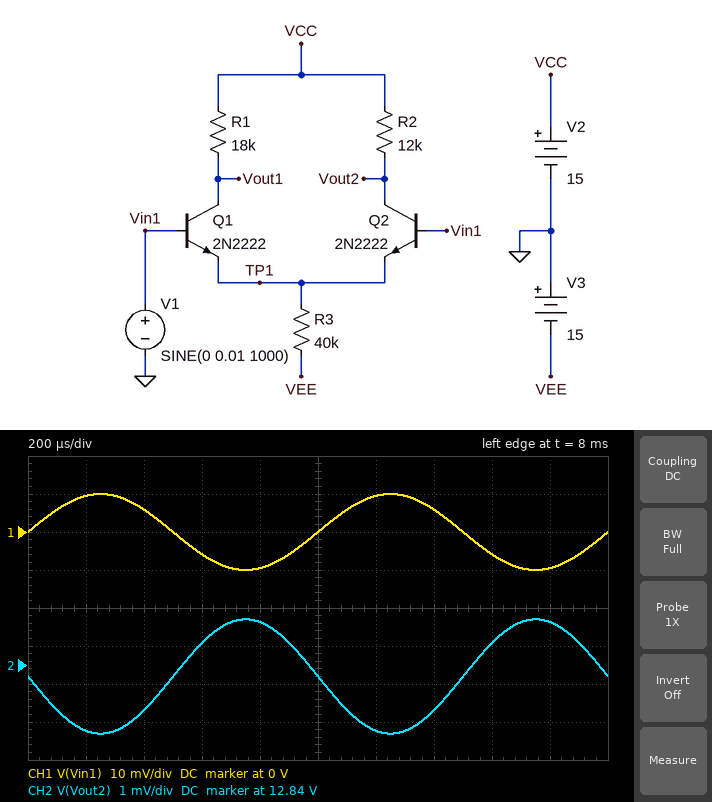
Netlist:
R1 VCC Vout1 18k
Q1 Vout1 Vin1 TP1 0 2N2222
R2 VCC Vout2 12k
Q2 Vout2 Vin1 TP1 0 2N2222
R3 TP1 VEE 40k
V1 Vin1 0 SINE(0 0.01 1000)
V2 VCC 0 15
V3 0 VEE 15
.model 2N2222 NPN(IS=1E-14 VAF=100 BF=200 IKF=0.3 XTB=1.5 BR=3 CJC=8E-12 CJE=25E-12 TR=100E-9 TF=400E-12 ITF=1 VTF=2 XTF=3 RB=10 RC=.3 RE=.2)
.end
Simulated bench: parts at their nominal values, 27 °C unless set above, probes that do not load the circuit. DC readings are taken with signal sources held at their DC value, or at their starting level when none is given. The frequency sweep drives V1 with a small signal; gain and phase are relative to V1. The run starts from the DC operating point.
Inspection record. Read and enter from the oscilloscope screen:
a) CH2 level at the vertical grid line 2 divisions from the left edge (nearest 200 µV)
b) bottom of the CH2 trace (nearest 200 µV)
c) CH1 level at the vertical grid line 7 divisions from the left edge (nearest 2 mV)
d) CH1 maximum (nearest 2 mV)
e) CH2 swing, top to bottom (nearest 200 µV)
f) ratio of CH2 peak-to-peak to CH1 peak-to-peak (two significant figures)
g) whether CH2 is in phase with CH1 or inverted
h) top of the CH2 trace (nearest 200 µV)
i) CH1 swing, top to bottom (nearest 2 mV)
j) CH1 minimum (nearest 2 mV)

12.8398 V
12.8392 V
6 mV
10 mV
3.0 mV
0.15
inverted
12.8422 V
20 mV
-10 mV
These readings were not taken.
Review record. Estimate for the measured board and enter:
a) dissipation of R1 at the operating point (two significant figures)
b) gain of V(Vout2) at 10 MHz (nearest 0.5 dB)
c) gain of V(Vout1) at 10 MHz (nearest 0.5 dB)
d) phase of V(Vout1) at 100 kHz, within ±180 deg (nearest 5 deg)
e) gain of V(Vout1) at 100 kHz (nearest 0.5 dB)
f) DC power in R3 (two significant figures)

570 µW
-0.5 dB
0 dB
170 deg
-13.0 dB
5.2 mW
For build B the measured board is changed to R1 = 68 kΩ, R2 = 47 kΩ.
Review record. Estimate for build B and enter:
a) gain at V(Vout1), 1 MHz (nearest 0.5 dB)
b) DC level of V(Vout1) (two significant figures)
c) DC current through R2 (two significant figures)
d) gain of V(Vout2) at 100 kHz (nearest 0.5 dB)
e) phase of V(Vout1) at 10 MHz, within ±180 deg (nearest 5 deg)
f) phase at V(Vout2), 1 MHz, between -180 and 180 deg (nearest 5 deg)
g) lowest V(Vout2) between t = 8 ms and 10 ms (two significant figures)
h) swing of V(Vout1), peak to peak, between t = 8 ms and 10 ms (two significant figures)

0 dB
3.0 V
180 µA
-4.5 dB
5 deg
70 deg
6.4 V
16 mV
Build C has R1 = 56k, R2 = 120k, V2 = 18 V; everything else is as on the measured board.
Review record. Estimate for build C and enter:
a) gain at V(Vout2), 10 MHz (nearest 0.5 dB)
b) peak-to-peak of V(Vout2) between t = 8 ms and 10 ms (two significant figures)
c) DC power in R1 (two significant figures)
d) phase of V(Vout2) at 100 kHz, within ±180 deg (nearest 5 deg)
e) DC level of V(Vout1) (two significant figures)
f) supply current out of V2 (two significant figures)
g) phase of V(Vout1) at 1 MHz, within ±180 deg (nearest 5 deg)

0 dB
19 mV
2.2 mW
0 deg
7.0 V
350 µA
70 deg
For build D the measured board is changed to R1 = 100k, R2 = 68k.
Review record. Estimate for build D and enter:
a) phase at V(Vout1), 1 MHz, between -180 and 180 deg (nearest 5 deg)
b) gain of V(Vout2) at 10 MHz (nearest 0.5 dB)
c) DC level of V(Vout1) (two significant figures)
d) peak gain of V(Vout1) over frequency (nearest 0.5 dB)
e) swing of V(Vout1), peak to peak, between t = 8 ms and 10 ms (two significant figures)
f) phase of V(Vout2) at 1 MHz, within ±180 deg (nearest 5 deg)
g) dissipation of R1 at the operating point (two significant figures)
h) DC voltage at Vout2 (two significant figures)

0 deg
0 dB
-560 mV
0 dB
19 mV
50 deg
2.4 mW
1.8 V
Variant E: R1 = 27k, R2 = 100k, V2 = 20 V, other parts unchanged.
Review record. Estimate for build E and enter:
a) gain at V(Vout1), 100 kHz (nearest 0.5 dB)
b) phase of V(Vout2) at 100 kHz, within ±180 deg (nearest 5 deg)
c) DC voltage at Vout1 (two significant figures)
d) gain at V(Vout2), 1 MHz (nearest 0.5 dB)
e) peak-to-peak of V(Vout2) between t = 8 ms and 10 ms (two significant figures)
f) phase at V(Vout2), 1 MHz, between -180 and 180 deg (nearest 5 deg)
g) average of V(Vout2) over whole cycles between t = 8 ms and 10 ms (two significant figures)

-8.5 dB
150 deg
15 V
0 dB
22 mV
40 deg
3.1 V
